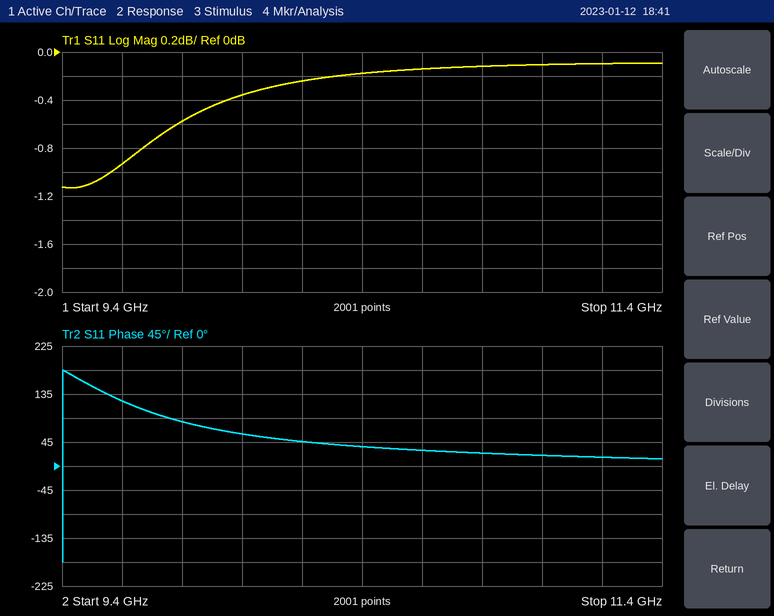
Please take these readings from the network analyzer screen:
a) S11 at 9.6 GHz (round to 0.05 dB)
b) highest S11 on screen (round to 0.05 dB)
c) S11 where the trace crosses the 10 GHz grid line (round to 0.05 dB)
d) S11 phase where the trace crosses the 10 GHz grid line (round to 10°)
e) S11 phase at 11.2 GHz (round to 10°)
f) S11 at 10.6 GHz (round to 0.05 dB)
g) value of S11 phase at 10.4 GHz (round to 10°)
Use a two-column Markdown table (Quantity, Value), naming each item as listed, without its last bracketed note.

| Quantity | Value |
|---|---|
| S11 at 9.6 GHz | -0.95 dB |
| highest S11 on screen | -0.10 dB |
| S11 where the trace crosses the 10 GHz grid line | -0.35 dB |
| S11 phase where the trace crosses the 10 GHz grid line | 60° |
| S11 phase at 11.2 GHz | 20° |
| S11 at 10.6 GHz | -0.15 dB |
| value of S11 phase at 10.4 GHz | 40° |
